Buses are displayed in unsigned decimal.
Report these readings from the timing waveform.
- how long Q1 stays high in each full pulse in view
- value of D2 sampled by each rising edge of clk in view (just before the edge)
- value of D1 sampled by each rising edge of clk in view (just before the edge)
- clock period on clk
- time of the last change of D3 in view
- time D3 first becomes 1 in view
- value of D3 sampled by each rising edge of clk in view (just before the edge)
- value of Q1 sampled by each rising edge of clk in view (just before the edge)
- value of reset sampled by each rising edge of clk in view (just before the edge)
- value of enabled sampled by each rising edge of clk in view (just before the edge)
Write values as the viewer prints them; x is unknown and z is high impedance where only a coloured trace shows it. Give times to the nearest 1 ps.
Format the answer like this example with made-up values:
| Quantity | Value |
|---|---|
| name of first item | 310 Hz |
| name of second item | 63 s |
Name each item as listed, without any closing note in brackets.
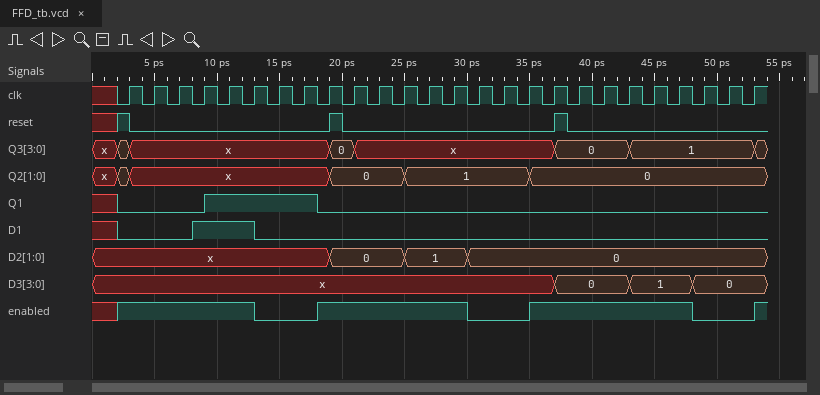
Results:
| Quantity | Value |
|---|---|
| how long Q1 stays high in each full pulse in view | 9 ps |
| value of D2 sampled by each rising edge of clk in view | x, x, x, x, x, x, x, x, x, 0, 0, 0, 1, 1, 0, 0, 0, 0, 0, 0, 0, 0, 0, 0, 0, 0 |
| value of D1 sampled by each rising edge of clk in view | 0 0 0 1 1 1 0 0 0 0 0 0 0 0 0 0 0 0 0 0 0 0 0 0 0 0 |
| clock period on clk | 2 ps |
| time of the last change of D3 in view | 48 ps |
| time D3 first becomes 1 in view | 43 ps |
| value of D3 sampled by each rising edge of clk in view | x, x, x, x, x, x, x, x, x, x, x, x, x, x, x, x, x, x, 0, 0, 0, 1, 1, 0, 0, 0 |
| value of Q1 sampled by each rising edge of clk in view | 0 0 0 0 1 1 1 1 0 0 0 0 0 0 0 0 0 0 0 0 0 0 0 0 0 0 |
| value of reset sampled by each rising edge of clk in view | 1 0 0 0 0 0 0 0 0 0 0 0 0 0 0 0 0 0 0 0 0 0 0 0 0 0 |
| value of enabled sampled by each rising edge of clk in view | 1 1 1 1 1 1 0 0 1 1 1 1 1 1 0 0 0 1 1 1 1 1 1 0 0 0 |
